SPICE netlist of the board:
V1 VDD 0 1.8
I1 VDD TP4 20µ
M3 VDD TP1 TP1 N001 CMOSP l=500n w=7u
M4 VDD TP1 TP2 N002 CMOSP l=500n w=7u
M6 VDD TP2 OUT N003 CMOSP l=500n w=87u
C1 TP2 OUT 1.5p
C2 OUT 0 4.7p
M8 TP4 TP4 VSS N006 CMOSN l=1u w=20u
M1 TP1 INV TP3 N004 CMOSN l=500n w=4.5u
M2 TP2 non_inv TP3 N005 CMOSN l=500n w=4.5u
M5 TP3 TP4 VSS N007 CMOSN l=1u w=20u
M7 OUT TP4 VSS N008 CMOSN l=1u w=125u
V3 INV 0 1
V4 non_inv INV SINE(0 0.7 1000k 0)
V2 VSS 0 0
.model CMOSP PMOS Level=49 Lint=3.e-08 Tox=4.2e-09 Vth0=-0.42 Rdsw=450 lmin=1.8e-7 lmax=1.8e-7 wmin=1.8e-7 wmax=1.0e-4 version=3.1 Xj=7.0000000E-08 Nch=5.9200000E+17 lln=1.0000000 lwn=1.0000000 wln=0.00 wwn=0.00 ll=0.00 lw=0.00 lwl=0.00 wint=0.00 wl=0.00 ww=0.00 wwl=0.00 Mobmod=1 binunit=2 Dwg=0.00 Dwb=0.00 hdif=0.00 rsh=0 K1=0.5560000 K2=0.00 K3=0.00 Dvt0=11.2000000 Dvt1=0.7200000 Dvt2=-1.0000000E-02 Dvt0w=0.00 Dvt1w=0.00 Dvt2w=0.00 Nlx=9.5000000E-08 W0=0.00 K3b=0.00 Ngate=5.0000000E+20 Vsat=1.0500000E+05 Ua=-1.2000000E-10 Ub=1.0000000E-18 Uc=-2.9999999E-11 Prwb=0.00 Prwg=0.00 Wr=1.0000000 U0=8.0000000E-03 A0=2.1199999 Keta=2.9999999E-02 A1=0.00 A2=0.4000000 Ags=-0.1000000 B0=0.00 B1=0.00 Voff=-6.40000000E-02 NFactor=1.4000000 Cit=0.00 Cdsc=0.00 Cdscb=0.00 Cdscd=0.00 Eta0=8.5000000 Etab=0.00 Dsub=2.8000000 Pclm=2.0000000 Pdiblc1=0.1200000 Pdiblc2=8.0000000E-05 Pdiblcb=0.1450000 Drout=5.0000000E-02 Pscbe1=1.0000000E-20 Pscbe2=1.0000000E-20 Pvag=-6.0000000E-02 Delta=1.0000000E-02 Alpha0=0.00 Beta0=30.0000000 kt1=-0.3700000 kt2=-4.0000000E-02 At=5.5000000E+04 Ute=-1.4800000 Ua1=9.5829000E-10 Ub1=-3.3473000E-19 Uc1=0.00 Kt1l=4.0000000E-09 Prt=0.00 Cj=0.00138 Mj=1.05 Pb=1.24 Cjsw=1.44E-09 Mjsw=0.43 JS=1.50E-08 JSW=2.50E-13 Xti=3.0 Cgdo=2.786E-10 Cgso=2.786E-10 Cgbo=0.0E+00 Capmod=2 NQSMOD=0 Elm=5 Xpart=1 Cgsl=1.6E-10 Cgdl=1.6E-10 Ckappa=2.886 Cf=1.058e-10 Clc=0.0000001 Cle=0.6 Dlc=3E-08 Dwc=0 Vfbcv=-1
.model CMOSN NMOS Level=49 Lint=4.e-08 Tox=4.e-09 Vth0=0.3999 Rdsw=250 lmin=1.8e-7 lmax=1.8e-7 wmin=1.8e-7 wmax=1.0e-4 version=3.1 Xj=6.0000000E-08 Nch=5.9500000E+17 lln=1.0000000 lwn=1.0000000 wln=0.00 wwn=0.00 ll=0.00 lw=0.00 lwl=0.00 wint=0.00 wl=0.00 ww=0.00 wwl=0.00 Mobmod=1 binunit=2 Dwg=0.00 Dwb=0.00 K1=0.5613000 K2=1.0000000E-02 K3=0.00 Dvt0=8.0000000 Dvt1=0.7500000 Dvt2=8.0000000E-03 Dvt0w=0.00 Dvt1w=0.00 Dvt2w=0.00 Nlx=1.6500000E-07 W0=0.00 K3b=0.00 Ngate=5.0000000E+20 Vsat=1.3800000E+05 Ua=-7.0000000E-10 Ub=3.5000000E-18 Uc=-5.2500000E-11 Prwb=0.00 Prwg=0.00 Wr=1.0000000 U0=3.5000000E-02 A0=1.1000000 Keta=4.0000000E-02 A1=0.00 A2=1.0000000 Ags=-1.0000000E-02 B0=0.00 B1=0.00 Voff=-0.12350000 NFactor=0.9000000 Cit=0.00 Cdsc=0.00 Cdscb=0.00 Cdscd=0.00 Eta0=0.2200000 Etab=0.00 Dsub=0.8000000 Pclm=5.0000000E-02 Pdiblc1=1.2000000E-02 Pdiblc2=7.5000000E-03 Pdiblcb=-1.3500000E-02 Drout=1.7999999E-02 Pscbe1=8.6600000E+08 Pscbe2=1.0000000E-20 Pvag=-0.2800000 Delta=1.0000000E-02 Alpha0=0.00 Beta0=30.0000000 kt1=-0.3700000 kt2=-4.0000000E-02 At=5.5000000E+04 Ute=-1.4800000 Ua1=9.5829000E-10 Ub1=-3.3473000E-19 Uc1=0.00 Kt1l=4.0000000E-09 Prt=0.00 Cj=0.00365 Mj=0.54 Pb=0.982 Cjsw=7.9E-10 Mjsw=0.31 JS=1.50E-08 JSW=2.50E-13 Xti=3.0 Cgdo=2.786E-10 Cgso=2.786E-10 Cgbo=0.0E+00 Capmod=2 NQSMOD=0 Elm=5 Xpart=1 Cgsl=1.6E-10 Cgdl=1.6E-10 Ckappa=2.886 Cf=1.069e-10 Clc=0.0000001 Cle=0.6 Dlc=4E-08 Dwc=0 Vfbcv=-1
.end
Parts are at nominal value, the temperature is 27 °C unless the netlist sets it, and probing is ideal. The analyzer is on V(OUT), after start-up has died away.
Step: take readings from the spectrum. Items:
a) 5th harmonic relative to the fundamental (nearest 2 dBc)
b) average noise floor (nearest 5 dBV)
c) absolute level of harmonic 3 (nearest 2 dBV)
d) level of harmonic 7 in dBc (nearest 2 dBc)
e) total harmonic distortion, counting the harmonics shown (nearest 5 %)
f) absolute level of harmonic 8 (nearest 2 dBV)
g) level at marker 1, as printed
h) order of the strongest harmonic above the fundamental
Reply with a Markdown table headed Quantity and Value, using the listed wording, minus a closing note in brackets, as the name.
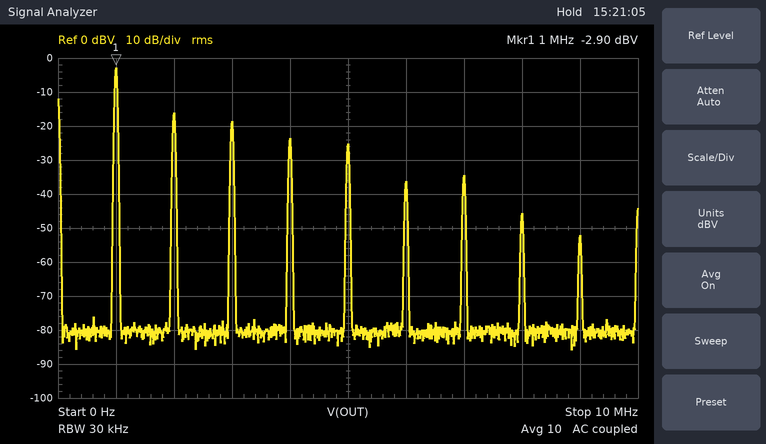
| Quantity | Value |
|---|---|
| 5th harmonic relative to the fundamental | -22 dBc |
| average noise floor | -80 dBV |
| absolute level of harmonic 3 | -18 dBV |
| level of harmonic 7 in dBc | -32 dBc |
| total harmonic distortion, counting the harmonics shown | 30 % |
| absolute level of harmonic 8 | -46 dBV |
| level at marker 1, as printed | -2.90 dBV |
| order of the strongest harmonic above the fundamental | 2 |
